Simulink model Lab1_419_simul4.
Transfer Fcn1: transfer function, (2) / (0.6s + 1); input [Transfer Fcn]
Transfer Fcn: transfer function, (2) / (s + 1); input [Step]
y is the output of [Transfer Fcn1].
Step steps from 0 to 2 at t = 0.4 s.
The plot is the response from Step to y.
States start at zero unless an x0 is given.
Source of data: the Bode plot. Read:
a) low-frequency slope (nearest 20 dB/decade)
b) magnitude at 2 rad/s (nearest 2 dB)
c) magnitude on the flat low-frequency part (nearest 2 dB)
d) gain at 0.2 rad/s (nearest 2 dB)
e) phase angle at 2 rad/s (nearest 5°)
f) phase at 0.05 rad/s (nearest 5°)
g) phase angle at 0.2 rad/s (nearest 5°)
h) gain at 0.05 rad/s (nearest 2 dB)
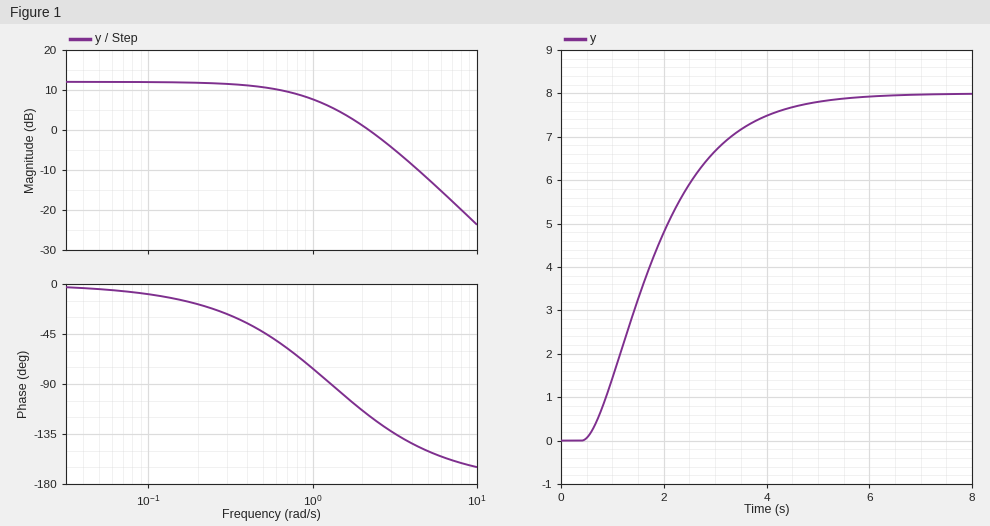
0 dB/decade
2 dB
12 dB
12 dB
-115°
-5°
-20°
12 dB
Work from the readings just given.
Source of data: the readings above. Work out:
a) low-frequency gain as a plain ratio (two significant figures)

4.0
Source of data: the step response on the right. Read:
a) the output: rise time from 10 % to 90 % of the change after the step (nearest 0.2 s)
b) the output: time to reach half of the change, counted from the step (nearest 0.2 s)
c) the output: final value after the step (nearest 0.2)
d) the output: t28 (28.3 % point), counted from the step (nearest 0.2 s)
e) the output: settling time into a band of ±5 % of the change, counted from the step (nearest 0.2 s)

2.8 s
1.4 s
8.0
0.8 s
3.8 s
